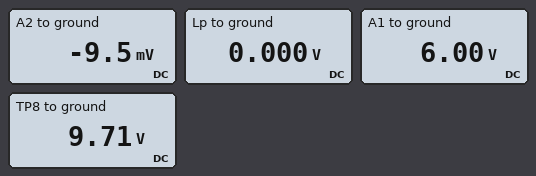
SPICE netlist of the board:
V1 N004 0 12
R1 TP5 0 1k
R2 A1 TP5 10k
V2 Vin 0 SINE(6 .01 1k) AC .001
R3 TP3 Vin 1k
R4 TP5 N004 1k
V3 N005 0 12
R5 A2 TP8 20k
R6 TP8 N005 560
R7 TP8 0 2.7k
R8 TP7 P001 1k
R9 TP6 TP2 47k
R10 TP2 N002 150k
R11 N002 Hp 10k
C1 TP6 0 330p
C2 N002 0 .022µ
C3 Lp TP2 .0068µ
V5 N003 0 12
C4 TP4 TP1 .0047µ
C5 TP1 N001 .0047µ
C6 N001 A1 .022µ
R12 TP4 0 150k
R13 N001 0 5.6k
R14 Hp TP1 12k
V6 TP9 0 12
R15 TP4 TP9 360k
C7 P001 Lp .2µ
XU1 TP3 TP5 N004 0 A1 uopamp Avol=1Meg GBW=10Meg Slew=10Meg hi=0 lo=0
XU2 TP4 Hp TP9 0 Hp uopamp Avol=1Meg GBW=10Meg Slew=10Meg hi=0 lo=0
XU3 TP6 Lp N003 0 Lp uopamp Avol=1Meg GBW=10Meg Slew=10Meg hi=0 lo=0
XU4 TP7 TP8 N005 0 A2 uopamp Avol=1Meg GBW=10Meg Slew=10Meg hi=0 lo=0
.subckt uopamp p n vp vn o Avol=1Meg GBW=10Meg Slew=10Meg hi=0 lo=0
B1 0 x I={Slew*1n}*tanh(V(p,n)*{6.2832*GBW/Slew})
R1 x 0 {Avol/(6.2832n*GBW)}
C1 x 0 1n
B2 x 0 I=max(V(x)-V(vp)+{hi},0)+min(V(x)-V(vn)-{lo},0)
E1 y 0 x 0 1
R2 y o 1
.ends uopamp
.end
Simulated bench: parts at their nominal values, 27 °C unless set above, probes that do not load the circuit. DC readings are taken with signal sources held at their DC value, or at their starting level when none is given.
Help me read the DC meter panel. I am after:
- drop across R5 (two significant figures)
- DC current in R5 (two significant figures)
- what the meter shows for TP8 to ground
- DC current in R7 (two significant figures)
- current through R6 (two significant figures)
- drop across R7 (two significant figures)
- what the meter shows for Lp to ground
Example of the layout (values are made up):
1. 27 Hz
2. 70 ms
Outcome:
1. 9.7 V
2. 490 µA
3. 9.71 V
4. 3.6 mA
5. 4.1 mA
6. 9.7 V
7. 0.000 V
